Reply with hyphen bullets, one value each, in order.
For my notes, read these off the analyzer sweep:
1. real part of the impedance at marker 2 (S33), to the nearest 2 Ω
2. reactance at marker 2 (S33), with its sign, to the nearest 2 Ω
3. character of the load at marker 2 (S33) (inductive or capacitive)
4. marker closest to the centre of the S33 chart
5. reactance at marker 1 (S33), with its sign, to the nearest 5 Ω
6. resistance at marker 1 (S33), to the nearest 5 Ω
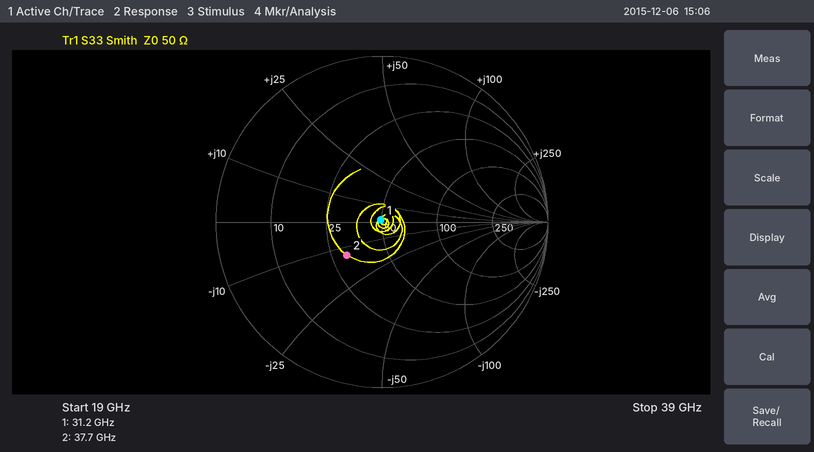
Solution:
- 30 Ω
- -14 Ω
- capacitive
- marker 1
- 0 Ω
- 50 Ω
